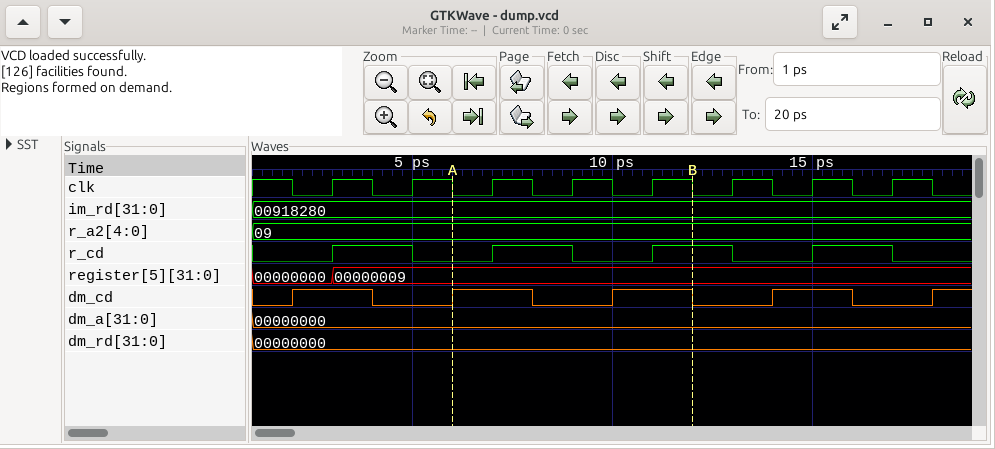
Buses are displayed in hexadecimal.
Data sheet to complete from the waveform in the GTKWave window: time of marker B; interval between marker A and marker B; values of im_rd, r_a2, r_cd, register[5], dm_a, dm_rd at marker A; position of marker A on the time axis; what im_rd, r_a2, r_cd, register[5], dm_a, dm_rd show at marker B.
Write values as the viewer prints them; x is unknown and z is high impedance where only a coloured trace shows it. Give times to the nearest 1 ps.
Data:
12 ps
6 ps
im_rd=00918280, r_a2=09, r_cd=0, register[5]=00000009, dm_a=00000000, dm_rd=00000000
6 ps
im_rd=00918280, r_a2=09, r_cd=1, register[5]=00000009, dm_a=00000000, dm_rd=00000000
